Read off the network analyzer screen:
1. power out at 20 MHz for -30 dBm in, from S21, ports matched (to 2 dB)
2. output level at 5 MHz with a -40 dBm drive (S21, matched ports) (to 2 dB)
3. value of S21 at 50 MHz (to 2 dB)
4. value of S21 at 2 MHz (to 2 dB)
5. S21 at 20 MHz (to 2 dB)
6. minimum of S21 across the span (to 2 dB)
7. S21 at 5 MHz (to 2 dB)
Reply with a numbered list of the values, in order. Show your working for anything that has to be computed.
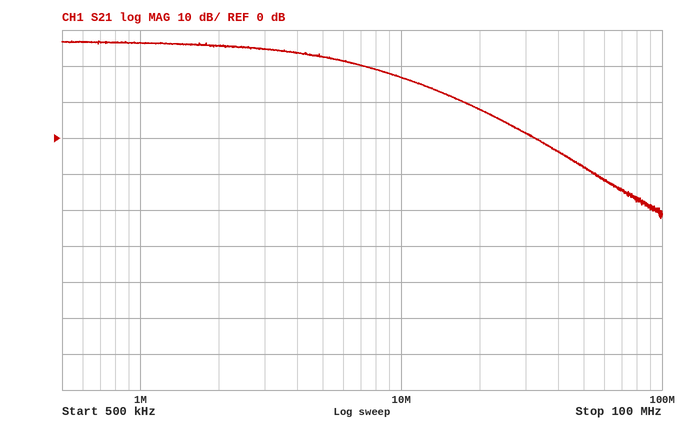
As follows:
1. -30 dBm + (8 dB) = -22 dBm
2. -40 dBm + (22 dB) = -18 dBm
3. -8 dB
4. 26 dB
5. 8 dB
6. -22 dB
7. 22 dB
